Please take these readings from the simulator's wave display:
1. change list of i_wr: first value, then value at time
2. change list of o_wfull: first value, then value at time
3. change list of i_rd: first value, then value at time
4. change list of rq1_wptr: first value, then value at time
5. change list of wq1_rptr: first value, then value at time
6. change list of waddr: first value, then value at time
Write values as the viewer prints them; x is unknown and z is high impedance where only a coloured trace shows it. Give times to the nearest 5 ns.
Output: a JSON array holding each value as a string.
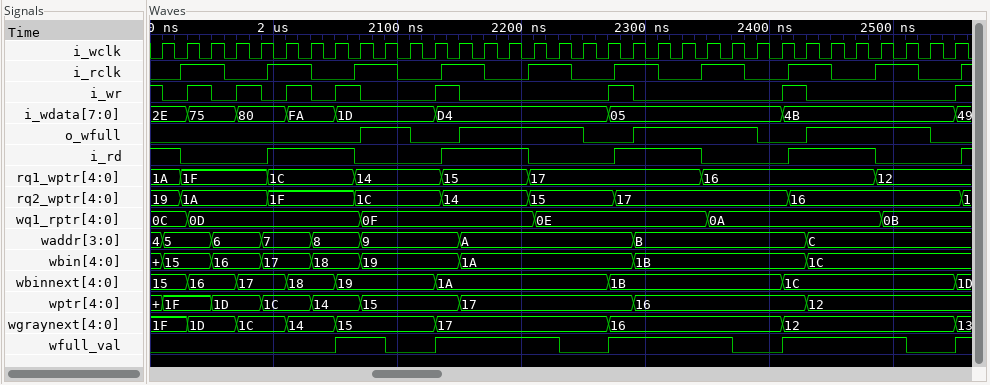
["1, 0 at 1910 ns, 1 at 1930 ns, 0 at 1950 ns, 1 at 1970 ns, 0 at 1990 ns, 1 at 2010 ns, 0 at 2030 ns, 1 at 2050 ns, 0 at 2070 ns, 1 at 2130 ns, 0 at 2150 ns, 1 at 2270 ns, 0 at 2290 ns, 1 at 2410 ns, 0 at 2430 ns, 1 at 2550 ns", "0, 1 at 2070 ns, 0 at 2110 ns, 1 at 2150 ns, 0 at 2250 ns, 1 at 2290 ns, 0 at 2390 ns, 1 at 2430 ns, 0 at 2530 ns", "1, 0 at 1925 ns, 1 at 1995 ns, 0 at 2065 ns, 1 at 2135 ns, 0 at 2205 ns, 1 at 2275 ns, 0 at 2345 ns, 1 at 2415 ns, 0 at 2485 ns, 1 at 2555 ns", "1A, 1F at 1925 ns, 1C at 1995 ns, 14 at 2065 ns, 15 at 2135 ns, 17 at 2205 ns, 16 at 2345 ns, 12 at 2485 ns", "0C, 0D at 1930 ns, 0F at 2070 ns, 0E at 2210 ns, 0A at 2350 ns, 0B at 2490 ns", "4, 5 at 1910 ns, 6 at 1950 ns, 7 at 1990 ns, 8 at 2030 ns, 9 at 2070 ns, A at 2150 ns, B at 2290 ns, C at 2430 ns"]
